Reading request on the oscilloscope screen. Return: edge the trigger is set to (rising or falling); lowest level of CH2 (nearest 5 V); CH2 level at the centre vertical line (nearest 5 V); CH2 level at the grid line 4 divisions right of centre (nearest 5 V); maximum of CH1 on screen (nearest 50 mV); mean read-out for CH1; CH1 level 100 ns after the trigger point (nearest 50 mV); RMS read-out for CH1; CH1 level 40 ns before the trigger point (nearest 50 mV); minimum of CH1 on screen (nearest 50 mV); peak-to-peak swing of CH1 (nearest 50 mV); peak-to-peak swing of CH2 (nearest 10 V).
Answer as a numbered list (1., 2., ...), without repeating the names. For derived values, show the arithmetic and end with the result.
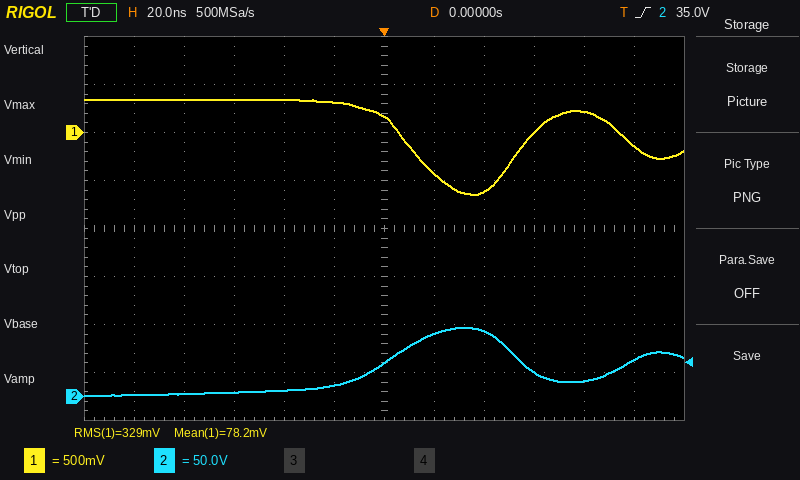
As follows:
1. rising
2. 0 V
3. 35 V
4. 15 V
5. 350 mV
6. 78.2 mV
7. -150 mV
8. 329 mV
9. 350 mV
10. -650 mV
11. 350 mV − (-650 mV) = 1.00 V
12. 70 V
